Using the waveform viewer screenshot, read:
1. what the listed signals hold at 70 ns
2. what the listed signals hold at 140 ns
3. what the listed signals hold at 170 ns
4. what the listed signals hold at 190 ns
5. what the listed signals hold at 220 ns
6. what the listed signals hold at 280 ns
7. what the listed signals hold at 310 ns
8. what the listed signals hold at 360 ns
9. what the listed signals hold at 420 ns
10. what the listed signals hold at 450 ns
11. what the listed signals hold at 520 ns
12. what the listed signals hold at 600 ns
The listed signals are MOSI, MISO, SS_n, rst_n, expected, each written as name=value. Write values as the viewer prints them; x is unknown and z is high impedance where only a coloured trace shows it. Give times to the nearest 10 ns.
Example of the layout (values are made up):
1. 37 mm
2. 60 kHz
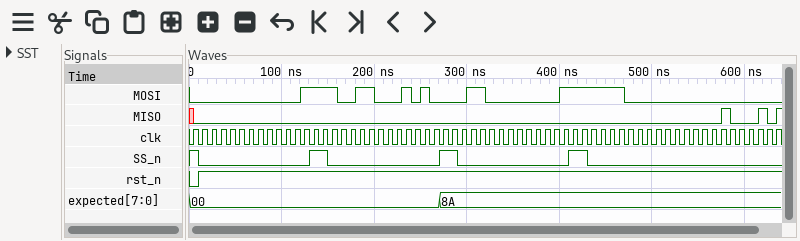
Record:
1. MOSI=0, MISO=0, SS_n=0, rst_n=1, expected=00
2. MOSI=1, MISO=0, SS_n=1, rst_n=1, expected=00
3. MOSI=0, MISO=0, SS_n=0, rst_n=1, expected=00
4. MOSI=1, MISO=0, SS_n=0, rst_n=1, expected=00
5. MOSI=0, MISO=0, SS_n=0, rst_n=1, expected=00
6. MOSI=0, MISO=0, SS_n=1, rst_n=1, expected=8A
7. MOSI=1, MISO=0, SS_n=0, rst_n=1, expected=8A
8. MOSI=0, MISO=0, SS_n=0, rst_n=1, expected=8A
9. MOSI=1, MISO=0, SS_n=1, rst_n=1, expected=8A
10. MOSI=1, MISO=0, SS_n=0, rst_n=1, expected=8A
11. MOSI=0, MISO=0, SS_n=0, rst_n=1, expected=8A
12. MOSI=0, MISO=0, SS_n=0, rst_n=1, expected=8A
